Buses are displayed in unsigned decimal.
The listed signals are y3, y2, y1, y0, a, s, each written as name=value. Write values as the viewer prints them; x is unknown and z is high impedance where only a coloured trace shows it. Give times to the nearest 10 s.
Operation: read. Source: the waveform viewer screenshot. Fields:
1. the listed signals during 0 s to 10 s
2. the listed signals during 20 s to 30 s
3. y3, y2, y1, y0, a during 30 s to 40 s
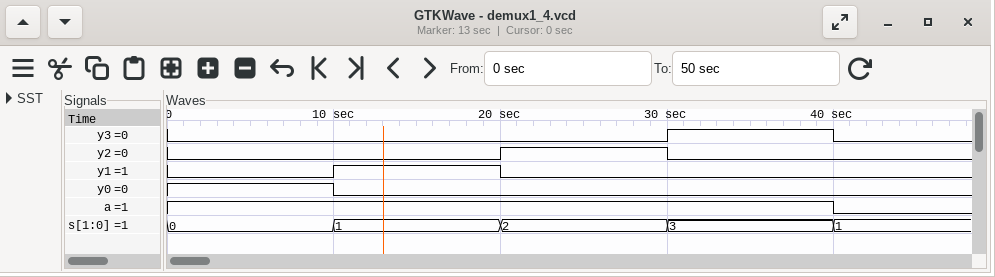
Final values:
y3=0, y2=0, y1=0, y0=1, a=1, s=0
y3=0, y2=1, y1=0, y0=0, a=1, s=2
y3=1, y2=0, y1=0, y0=0, a=1
